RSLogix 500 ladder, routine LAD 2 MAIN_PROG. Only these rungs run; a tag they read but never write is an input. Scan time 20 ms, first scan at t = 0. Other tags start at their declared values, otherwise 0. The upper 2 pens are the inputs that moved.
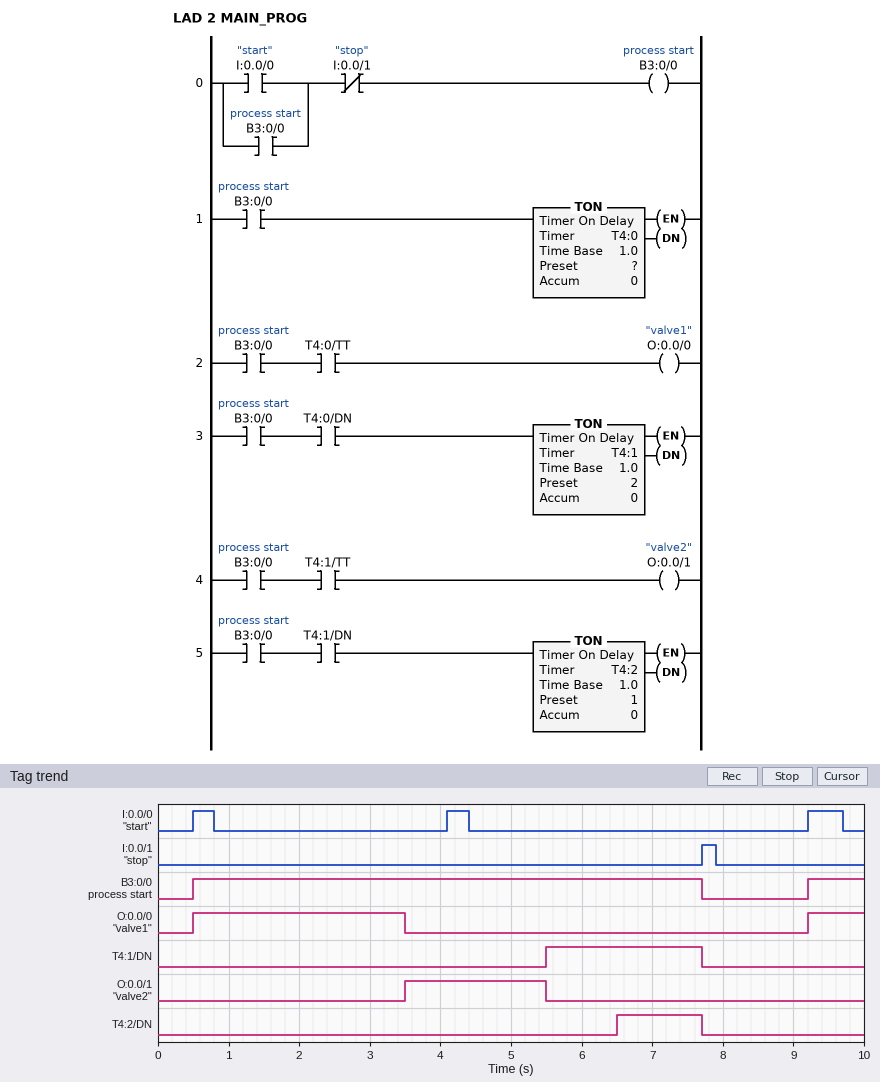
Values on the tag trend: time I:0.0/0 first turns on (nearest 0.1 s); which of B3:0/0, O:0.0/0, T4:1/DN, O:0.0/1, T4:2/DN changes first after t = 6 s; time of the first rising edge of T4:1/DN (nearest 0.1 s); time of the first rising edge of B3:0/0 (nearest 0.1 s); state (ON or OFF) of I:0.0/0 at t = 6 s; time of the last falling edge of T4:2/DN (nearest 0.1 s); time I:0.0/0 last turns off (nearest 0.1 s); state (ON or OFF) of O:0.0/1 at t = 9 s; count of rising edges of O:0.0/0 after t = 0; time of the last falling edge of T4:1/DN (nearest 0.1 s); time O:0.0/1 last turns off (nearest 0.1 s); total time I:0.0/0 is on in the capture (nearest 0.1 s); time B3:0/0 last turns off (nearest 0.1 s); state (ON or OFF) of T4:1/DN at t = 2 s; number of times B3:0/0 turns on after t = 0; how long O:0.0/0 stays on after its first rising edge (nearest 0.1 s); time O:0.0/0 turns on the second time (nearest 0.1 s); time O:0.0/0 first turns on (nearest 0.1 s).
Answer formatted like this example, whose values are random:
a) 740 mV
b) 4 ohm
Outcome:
a) 0.5 s
b) T4:2/DN
c) 5.5 s
d) 0.5 s
e) OFF
f) 7.7 s
g) 9.7 s
h) OFF
i) 2
j) 7.7 s
k) 5.5 s
l) 1.1 s
m) 7.7 s
n) OFF
o) 2
p) 3.0 s
q) 9.2 s
r) 0.5 s
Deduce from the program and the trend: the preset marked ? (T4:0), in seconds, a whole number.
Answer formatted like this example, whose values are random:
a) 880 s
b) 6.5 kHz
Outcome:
a) 3 s
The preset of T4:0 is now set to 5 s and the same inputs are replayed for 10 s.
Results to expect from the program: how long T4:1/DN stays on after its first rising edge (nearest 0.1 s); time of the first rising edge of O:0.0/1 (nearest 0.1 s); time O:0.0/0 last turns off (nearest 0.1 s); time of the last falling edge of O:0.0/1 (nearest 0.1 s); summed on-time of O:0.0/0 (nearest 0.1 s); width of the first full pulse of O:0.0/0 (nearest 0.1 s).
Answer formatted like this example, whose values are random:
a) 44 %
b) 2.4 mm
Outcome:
a) 0.2 s
b) 5.5 s
c) 5.5 s
d) 7.5 s
e) 5.8 s
f) 5.0 s
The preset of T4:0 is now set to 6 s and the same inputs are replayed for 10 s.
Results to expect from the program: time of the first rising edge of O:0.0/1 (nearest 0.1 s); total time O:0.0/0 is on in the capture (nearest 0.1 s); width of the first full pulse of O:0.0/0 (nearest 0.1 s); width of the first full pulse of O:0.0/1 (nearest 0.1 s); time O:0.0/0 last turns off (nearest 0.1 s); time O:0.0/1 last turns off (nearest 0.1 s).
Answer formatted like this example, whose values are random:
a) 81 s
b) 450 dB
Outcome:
a) 6.5 s
b) 6.8 s
c) 6.0 s
d) 1.2 s
e) 6.5 s
f) 7.7 s
